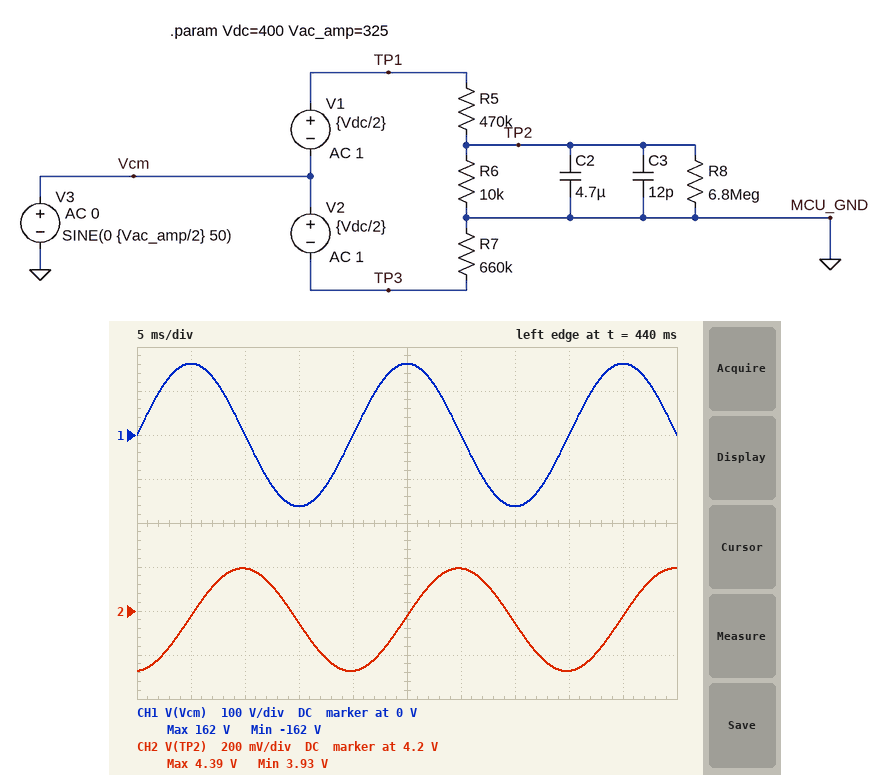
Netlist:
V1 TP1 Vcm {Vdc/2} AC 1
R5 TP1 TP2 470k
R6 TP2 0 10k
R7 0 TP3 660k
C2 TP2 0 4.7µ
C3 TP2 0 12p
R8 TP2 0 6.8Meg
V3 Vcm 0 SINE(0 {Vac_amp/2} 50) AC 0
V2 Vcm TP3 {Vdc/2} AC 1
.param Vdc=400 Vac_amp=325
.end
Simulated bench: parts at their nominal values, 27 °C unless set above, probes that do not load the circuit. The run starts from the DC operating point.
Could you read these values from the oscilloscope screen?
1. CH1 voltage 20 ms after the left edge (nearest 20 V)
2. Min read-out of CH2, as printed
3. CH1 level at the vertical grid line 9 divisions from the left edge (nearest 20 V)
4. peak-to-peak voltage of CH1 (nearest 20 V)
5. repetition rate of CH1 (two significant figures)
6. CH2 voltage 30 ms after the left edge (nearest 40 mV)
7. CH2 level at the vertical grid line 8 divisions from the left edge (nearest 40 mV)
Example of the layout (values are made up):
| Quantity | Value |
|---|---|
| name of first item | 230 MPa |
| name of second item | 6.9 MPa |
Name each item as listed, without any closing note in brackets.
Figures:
| Quantity | Value |
|---|---|
| CH1 voltage 20 ms after the left edge | 0 V |
| Min read-out of CH2, as printed | 3.93 V |
| CH1 level at the vertical grid line 9 divisions from the left edge | 160 V |
| peak-to-peak voltage of CH1 | 320 V |
| repetition rate of CH1 | 50 Hz |
| CH2 voltage 30 ms after the left edge | 4.40 V |
| CH2 level at the vertical grid line 8 divisions from the left edge | 3.92 V |
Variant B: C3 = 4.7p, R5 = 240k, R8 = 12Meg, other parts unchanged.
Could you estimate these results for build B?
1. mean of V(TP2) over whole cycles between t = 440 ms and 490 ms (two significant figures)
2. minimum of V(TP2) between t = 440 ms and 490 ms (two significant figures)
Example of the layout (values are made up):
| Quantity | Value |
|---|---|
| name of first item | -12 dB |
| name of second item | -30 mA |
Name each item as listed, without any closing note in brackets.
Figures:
| Quantity | Value |
|---|---|
| mean of V(TP2) over whole cycles between t = 440 ms and 490 ms | 8.0 V |
| minimum of V(TP2) between t = 440 ms and 490 ms | 7.5 V |
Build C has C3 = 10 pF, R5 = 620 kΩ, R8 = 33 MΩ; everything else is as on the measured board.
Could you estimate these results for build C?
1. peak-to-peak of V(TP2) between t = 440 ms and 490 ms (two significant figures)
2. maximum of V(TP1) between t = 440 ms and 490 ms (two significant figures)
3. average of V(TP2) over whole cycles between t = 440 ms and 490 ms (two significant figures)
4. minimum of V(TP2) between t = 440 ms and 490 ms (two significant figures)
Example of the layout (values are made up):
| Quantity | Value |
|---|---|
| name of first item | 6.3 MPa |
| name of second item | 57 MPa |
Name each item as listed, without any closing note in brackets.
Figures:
| Quantity | Value |
|---|---|
| peak-to-peak of V(TP2) between t = 440 ms and 490 ms | 350 mV |
| maximum of V(TP1) between t = 440 ms and 490 ms | 360 V |
| average of V(TP2) over whole cycles between t = 440 ms and 490 ms | 3.2 V |
| minimum of V(TP2) between t = 440 ms and 490 ms | 3.0 V |
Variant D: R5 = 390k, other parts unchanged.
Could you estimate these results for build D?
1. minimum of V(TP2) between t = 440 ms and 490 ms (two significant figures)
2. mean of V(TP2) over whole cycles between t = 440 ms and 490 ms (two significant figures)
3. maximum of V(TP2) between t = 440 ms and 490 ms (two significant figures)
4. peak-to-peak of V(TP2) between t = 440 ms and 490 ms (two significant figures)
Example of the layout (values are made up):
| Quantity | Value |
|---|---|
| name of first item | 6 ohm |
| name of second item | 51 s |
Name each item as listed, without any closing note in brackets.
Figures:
| Quantity | Value |
|---|---|
| minimum of V(TP2) between t = 440 ms and 490 ms | 4.7 V |
| mean of V(TP2) over whole cycles between t = 440 ms and 490 ms | 5.0 V |
| maximum of V(TP2) between t = 440 ms and 490 ms | 5.3 V |
| peak-to-peak of V(TP2) between t = 440 ms and 490 ms | 560 mV |
